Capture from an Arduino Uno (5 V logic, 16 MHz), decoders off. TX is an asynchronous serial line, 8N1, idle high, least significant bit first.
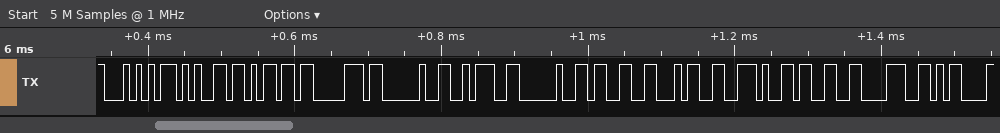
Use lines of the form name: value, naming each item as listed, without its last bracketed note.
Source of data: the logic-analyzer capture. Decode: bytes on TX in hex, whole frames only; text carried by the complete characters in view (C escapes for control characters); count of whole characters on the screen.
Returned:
bytes on TX in hex, whole frames only: 54 65 6D 70 20 3A 20 33 34 2E 33 38 0D
text carried by the complete characters in view: "Temp : 34.38\r"
count of whole characters on the screen: 13
